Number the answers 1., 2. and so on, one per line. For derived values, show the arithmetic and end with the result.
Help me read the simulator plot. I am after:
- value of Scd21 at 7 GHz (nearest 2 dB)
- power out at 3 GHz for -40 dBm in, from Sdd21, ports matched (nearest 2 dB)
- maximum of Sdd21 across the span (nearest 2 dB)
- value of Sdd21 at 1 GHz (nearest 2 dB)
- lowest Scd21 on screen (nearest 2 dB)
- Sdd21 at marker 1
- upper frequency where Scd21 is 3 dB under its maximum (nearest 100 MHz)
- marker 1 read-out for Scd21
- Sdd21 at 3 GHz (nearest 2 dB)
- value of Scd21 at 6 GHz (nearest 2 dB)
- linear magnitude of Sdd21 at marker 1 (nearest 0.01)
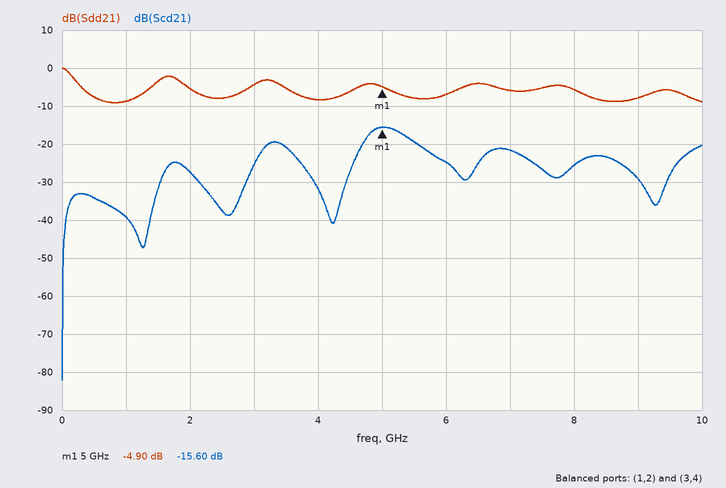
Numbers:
1. -22 dB
2. -40 dBm + (-4 dB) = -44 dBm
3. 0 dB
4. -8 dB
5. -82 dB
6. -4.90 dB
7. 5.4 GHz
8. -15.60 dB
9. -4 dB
10. -24 dB
11. 10^(-4.9/20) ≈ 0.57
